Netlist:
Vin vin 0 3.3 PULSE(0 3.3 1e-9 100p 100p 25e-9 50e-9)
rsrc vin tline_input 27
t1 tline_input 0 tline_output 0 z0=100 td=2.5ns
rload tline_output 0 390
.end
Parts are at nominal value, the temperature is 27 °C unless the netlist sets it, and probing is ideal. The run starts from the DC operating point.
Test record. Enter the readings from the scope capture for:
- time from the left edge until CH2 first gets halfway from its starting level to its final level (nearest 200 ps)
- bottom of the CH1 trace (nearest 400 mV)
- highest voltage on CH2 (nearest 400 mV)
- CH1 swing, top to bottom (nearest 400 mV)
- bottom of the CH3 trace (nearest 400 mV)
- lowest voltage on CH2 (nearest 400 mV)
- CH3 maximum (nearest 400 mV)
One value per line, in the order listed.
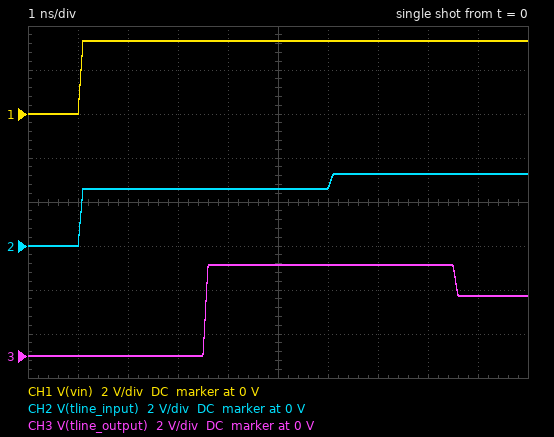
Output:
1.0 ns
0 V
3.2 V
3.2 V
0 V
0 V
4.0 V
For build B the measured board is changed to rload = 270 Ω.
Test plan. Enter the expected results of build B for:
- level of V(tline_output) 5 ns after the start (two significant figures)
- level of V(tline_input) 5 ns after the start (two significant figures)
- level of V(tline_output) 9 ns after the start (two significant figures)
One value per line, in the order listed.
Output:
3.8 V
2.6 V
2.8 V
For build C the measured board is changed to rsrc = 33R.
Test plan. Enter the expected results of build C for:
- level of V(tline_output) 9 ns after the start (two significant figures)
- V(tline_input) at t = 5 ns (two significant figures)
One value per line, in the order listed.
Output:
2.8 V
2.5 V
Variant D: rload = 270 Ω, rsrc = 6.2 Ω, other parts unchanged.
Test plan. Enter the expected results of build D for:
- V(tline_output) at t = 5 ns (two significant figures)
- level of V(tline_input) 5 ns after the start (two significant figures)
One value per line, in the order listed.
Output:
4.5 V
3.1 V
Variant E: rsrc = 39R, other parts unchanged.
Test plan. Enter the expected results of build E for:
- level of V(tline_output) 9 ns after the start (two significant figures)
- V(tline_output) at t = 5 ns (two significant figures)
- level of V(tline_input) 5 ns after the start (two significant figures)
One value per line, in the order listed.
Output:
2.8 V
3.8 V
2.4 V
